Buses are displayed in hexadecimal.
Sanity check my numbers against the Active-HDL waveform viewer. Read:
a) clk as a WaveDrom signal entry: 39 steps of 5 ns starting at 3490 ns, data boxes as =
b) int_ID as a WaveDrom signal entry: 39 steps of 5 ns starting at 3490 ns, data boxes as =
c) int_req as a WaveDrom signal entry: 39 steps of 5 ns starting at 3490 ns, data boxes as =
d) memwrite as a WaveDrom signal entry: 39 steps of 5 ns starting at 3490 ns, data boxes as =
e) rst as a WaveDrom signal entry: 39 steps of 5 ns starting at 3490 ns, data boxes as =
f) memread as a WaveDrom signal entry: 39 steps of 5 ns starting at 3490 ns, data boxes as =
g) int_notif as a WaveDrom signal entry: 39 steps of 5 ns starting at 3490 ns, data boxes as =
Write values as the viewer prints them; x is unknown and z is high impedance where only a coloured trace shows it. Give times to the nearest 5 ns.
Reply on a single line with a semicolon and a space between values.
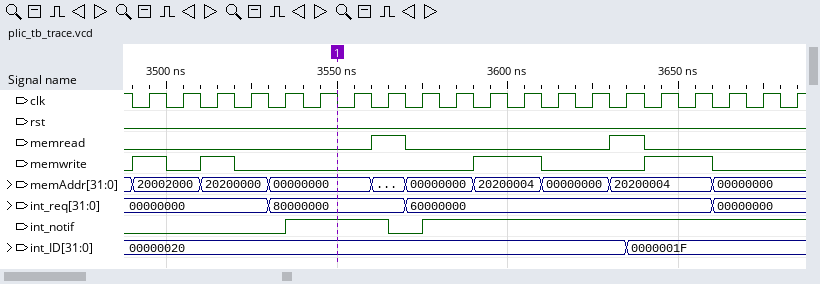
{name: 'clk', wave: '010101010101010101010101010101010101010'}; {name: 'int_ID', wave: '=............................=.........', data: '00000020 0000001F'}; {name: 'int_req', wave: '=.......=.......=.................=....', data: '00000000 80000000 60000000 00000000'}; {name: 'memwrite', wave: '1.0.1.0.............1...0.....1...0....'}; {name: 'rst', wave: '0......................................'}; {name: 'memread', wave: '0.............1.0...........1.0........'}; {name: 'int_notif', wave: '0........1.....0.1.....................'}
